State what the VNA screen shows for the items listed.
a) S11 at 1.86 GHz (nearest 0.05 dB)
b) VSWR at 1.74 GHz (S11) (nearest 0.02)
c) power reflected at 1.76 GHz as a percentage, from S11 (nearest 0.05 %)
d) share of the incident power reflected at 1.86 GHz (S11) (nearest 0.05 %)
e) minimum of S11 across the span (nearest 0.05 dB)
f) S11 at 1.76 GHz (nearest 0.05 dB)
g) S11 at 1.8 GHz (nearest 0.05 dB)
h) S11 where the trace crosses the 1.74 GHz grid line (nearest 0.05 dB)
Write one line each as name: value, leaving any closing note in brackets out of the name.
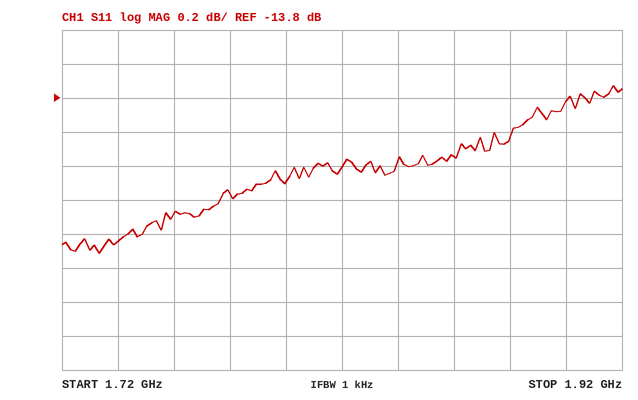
S11 at 1.86 GHz: -14.15 dB
VSWR at 1.74 GHz (S11): 1.46
power reflected at 1.76 GHz as a percentage, from S11: 3.55 %
share of the incident power reflected at 1.86 GHz (S11): 3.85 %
minimum of S11 across the span: -14.70 dB
S11 at 1.76 GHz: -14.50 dB
S11 at 1.8 GHz: -14.30 dB
S11 where the trace crosses the 1.74 GHz grid line: -14.65 dB
